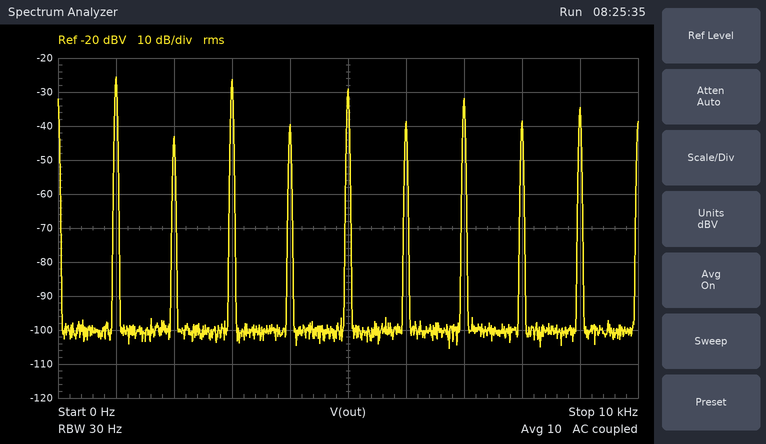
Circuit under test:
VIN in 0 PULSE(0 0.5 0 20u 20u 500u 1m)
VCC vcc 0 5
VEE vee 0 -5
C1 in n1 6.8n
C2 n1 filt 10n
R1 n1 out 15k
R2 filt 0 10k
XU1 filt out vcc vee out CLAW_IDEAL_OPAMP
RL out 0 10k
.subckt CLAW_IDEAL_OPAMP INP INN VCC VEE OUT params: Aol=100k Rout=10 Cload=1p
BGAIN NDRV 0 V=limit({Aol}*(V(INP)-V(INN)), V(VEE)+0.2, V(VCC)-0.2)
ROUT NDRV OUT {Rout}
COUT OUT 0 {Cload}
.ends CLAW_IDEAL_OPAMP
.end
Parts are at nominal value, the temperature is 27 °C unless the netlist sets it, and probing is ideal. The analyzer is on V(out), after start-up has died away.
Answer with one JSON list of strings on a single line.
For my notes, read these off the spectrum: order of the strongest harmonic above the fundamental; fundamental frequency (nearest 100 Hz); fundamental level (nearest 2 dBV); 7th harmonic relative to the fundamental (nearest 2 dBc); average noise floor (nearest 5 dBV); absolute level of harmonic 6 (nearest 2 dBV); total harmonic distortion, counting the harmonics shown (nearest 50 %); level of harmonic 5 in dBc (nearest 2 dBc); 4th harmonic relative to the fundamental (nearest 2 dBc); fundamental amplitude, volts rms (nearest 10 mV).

["3", "1.0 kHz", "-26 dBV", "-6 dBc", "-100 dBV", "-38 dBV", "150 %", "-4 dBc", "-14 dBc", "50 mV"]
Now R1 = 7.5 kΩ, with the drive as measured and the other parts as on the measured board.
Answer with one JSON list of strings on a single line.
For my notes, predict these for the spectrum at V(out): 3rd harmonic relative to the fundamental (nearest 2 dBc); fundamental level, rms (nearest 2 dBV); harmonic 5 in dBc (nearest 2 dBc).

["2 dBc", "-28 dBV", "0 dBc"]
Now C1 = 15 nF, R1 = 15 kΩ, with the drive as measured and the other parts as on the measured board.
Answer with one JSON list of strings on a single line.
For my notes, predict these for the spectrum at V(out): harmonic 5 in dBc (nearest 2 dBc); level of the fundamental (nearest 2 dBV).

["-6 dBc", "-22 dBV"]
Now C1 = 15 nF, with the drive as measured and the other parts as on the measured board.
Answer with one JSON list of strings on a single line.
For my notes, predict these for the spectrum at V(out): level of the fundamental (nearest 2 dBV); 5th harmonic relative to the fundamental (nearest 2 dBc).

["-22 dBV", "-6 dBc"]
